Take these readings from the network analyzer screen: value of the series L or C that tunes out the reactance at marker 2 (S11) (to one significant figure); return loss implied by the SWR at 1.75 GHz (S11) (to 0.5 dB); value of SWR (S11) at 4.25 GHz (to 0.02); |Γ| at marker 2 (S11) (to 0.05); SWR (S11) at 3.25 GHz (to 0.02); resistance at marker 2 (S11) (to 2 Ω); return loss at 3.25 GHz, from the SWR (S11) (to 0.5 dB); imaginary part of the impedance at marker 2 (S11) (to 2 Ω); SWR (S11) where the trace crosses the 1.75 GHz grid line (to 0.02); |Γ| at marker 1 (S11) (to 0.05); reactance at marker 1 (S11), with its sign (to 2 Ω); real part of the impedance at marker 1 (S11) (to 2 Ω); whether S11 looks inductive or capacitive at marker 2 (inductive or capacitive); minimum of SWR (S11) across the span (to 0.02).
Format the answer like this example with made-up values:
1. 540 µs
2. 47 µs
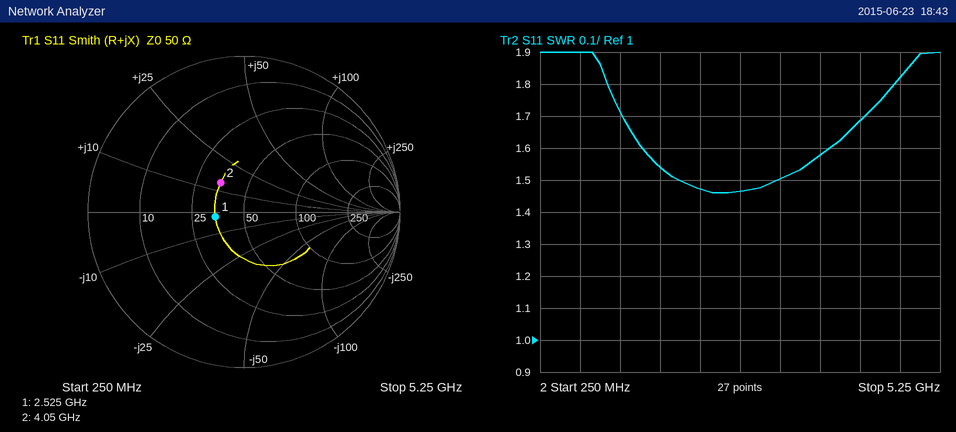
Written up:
1. 3 pF
2. 13.5 dB
3. 1.68
4. 0.25
5. 1.50
6. 34 Ω
7. 14.0 dB
8. +14 Ω
9. 1.54
10. 0.20
11. -2 Ω
12. 34 Ω
13. inductive
14. 1.46
